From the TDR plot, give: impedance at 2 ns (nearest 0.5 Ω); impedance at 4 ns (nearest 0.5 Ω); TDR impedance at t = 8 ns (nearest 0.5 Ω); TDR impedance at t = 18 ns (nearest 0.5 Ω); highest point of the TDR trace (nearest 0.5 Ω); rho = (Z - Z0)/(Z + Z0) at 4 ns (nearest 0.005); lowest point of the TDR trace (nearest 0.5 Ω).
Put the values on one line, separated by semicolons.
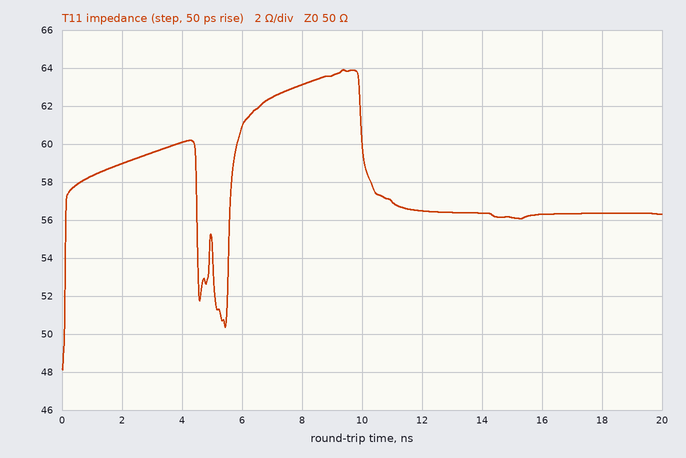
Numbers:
59.0 Ω; 60.0 Ω; 63.0 Ω; 56.5 Ω; 64.0 Ω; +0.090; 48.0 Ω
